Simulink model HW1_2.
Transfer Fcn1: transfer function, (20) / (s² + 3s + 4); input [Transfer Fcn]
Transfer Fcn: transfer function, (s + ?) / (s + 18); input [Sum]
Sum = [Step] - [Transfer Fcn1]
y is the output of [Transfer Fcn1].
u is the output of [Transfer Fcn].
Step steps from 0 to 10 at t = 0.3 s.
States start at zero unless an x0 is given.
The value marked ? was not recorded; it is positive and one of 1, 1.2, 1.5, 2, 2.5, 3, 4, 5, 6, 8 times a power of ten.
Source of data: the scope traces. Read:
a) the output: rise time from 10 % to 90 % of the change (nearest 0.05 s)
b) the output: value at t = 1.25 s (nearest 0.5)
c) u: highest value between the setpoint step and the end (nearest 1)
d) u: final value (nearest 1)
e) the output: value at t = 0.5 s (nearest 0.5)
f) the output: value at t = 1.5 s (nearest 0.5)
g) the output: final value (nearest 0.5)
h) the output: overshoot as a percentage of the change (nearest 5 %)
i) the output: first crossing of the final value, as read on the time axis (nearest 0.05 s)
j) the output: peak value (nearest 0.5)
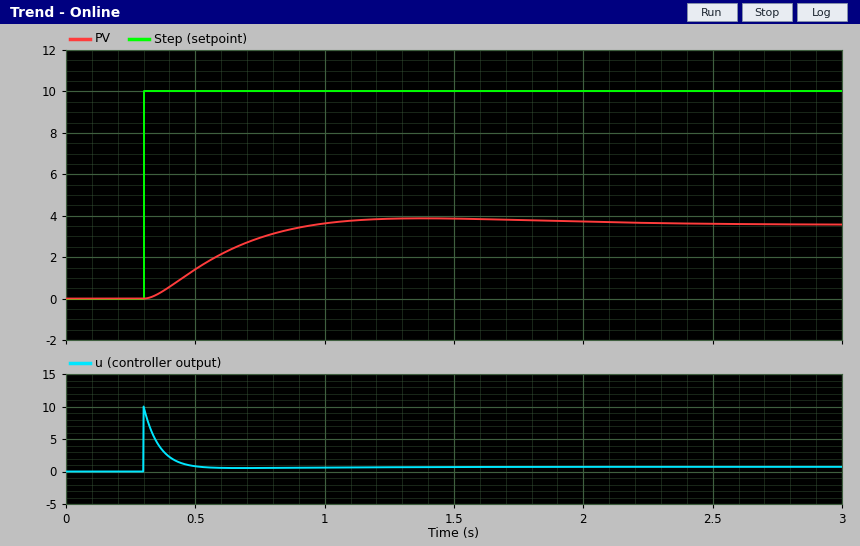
0.45 s
4.0
10
1
1.5
4.0
3.5
10 %
0.95 s
4.0
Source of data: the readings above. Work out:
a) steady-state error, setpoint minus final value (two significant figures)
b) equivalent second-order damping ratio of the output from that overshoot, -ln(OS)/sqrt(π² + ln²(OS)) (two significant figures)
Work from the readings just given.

6.5
0.59
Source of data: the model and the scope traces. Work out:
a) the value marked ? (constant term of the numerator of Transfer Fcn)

2
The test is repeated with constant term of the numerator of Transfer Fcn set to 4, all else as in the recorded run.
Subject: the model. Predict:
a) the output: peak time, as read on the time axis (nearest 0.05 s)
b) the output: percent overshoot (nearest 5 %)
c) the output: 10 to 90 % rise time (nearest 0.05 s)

1.40 s
10 %
0.50 s
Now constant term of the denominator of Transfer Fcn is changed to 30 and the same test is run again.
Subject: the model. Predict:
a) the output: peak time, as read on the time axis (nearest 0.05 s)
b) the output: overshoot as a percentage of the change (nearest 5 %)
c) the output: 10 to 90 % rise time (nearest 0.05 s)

1.50 s
10 %
0.50 s
